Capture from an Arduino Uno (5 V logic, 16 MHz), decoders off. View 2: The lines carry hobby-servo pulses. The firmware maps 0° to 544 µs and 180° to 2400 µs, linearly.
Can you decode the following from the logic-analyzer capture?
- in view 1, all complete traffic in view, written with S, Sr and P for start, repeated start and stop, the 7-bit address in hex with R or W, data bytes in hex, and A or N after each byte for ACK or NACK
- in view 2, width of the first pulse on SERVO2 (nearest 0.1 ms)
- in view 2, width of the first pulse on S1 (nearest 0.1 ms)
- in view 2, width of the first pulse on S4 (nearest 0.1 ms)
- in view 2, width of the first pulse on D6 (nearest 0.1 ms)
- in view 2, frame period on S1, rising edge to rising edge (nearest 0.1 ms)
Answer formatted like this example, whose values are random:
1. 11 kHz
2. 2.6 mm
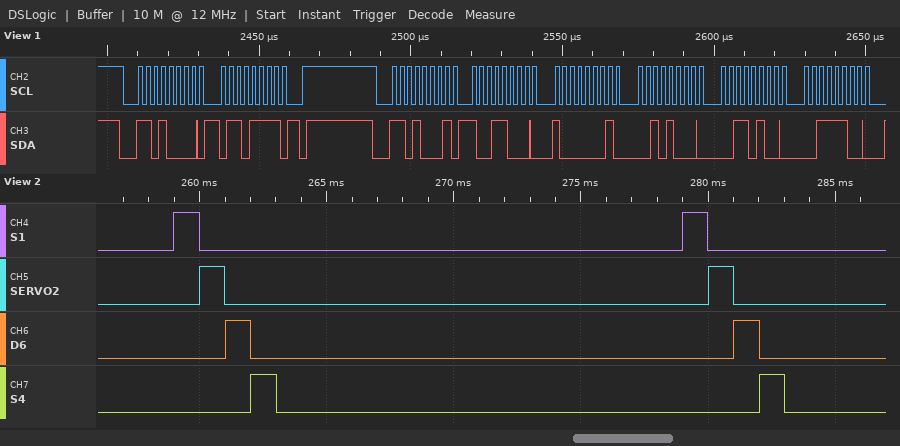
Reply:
1. S 68W A 6F A P S 68R A 98 A 81 A 28 A 34 A 3C A
2. 1.0 ms
3. 1.0 ms
4. 1.0 ms
5. 1.0 ms
6. 20.0 ms
